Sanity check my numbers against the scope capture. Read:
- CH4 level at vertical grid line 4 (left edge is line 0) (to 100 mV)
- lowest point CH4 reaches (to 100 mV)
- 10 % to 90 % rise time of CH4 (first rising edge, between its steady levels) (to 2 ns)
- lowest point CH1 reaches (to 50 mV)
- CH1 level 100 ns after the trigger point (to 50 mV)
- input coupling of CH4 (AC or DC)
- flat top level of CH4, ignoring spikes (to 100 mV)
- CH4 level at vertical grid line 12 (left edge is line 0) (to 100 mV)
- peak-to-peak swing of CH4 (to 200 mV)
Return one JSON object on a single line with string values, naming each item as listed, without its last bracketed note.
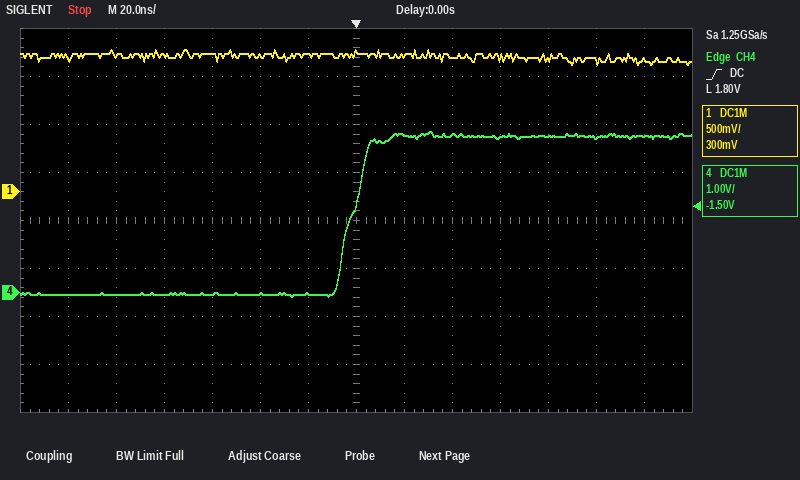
{"CH4 level at vertical grid line 4 (left edge is line 0)": "0.0 V", "lowest point CH4 reaches": "-100 mV", "10 % to 90 % rise time of CH4 (first rising edge, between its steady levels)": "12 ns", "lowest point CH1 reaches": "1.30 V", "CH1 level 100 ns after the trigger point": "1.35 V", "input coupling of CH4": "DC", "flat top level of CH4, ignoring spikes": "3.3 V", "CH4 level at vertical grid line 12 (left edge is line 0)": "3.2 V", "peak-to-peak swing of CH4": "3.4 V"}
